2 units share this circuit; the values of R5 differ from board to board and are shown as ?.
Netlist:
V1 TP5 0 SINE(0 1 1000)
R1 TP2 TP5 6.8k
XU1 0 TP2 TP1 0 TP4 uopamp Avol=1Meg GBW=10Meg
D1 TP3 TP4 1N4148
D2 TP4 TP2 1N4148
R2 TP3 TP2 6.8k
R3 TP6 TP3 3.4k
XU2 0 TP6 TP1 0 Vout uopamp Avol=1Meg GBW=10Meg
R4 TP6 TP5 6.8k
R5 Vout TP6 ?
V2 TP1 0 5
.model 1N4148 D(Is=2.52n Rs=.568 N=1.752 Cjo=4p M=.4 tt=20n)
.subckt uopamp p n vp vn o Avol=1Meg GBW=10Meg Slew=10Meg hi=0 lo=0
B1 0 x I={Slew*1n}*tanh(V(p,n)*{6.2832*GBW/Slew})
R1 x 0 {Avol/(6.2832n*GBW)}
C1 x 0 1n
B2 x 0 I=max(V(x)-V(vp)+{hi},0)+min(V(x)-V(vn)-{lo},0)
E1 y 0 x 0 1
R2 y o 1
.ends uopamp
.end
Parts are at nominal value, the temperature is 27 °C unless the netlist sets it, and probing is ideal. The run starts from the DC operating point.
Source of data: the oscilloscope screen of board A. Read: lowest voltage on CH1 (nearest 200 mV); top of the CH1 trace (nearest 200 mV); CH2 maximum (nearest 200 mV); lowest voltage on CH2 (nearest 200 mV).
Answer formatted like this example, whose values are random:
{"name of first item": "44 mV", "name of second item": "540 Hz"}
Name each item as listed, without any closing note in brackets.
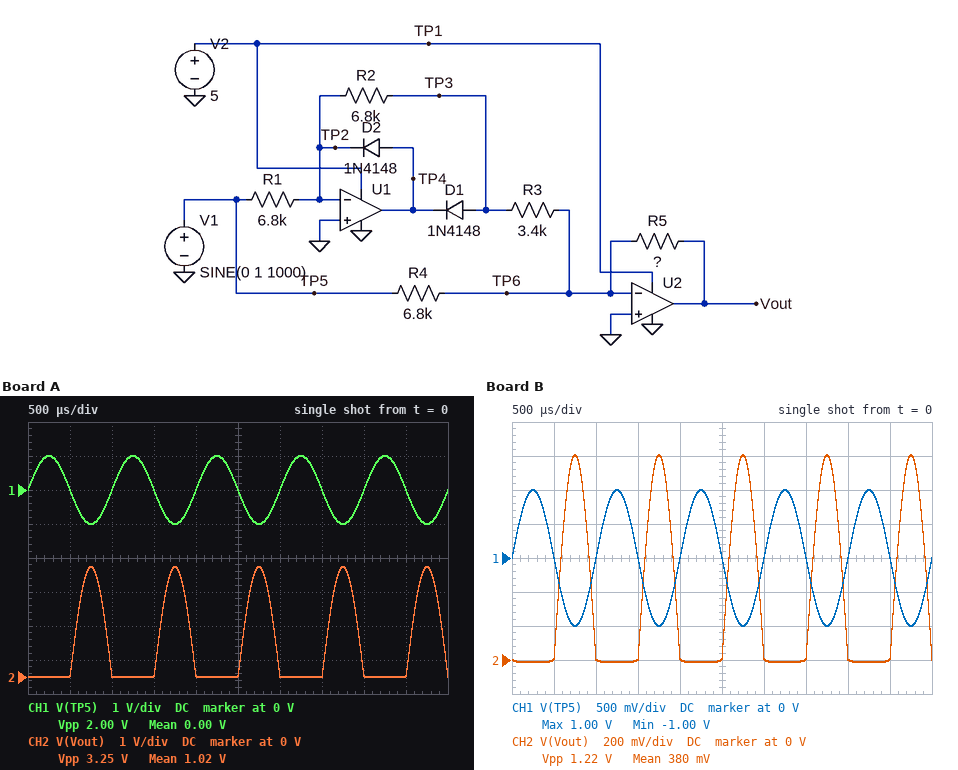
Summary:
{"lowest voltage on CH1": "-1.0 V", "top of the CH1 trace": "1.0 V", "CH2 maximum": "3.2 V", "lowest voltage on CH2": "0 V"}
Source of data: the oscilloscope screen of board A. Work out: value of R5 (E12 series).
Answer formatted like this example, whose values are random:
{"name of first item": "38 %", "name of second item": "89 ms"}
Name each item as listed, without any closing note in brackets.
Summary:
{"value of R5": "22 kΩ"}
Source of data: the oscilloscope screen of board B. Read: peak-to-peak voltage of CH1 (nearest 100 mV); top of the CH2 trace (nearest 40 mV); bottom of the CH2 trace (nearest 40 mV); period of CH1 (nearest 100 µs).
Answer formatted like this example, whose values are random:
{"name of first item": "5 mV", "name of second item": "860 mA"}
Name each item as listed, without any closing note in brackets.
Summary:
{"peak-to-peak voltage of CH1": "2.0 V", "top of the CH2 trace": "1.20 V", "bottom of the CH2 trace": "0 V", "period of CH1": "1.0 ms"}
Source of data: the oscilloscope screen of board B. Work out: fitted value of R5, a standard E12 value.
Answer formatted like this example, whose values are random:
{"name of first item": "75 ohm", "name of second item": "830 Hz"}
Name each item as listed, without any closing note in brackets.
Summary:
{"fitted value of R5, a standard E12 value": "8.2 kΩ"}
